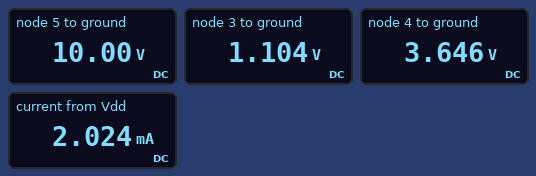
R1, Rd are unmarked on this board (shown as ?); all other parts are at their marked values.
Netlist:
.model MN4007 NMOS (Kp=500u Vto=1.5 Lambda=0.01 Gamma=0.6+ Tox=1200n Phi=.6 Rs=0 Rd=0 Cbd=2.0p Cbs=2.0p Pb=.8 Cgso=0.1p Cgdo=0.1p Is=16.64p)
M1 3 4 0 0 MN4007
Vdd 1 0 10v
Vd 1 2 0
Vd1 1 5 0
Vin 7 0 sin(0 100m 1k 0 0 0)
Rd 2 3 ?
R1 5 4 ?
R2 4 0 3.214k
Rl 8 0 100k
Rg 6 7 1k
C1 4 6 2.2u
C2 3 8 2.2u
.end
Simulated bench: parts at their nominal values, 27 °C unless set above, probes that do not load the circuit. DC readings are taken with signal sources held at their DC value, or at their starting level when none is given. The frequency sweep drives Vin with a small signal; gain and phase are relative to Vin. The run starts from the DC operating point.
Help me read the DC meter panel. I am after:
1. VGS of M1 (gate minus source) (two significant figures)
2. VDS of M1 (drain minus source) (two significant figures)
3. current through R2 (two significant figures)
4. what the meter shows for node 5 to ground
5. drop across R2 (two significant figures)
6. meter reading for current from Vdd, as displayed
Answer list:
3.6 V
1.1 V
1.1 mA
10.00 V
3.6 V
2.024 mA
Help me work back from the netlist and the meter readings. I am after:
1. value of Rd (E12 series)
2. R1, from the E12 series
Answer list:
10 kΩ
5.6 kΩ
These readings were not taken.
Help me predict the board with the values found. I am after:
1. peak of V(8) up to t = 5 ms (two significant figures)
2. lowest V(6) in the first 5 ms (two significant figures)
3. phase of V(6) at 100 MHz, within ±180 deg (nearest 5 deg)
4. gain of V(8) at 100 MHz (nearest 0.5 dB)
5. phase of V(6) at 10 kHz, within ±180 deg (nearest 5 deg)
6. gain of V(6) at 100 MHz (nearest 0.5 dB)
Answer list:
64 mV
-67 mV
-5 deg
-9.5 dB
0 deg
-3.5 dB
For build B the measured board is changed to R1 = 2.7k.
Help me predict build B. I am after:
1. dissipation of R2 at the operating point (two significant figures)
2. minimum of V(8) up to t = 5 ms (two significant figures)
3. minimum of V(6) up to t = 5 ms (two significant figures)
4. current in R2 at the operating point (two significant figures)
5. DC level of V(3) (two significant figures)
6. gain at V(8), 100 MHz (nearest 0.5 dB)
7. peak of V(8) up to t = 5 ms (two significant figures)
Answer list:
9.2 mW
-8.1 mV
-59 mV
1.7 mA
510 mV
-22.5 dB
8.7 mV
